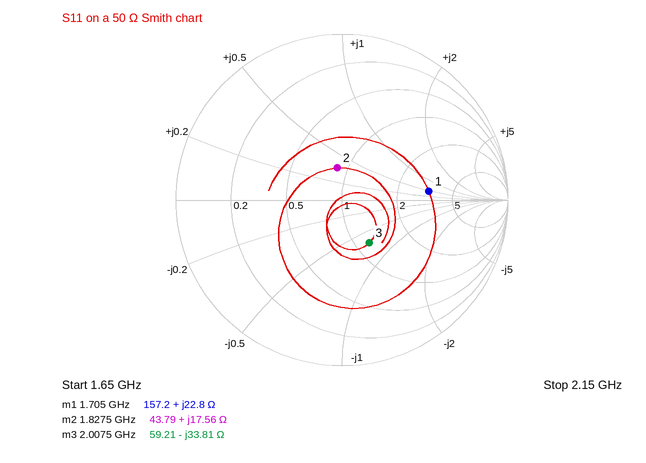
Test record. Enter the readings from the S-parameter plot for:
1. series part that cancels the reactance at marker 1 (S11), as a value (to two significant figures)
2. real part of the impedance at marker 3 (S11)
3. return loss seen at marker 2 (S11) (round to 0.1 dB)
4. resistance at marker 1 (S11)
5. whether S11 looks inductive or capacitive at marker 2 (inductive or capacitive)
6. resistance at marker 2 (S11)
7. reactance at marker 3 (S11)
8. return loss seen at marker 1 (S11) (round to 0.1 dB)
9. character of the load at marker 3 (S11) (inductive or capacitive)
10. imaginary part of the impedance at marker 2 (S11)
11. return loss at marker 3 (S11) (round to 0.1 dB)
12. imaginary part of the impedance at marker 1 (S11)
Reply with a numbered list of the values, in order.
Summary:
1. 4.1 pF
2. 59.21 Ω
3. 14.2 dB
4. 157.2 Ω
5. inductive
6. 43.79 Ω
7. -33.81 Ω
8. 5.6 dB
9. capacitive
10. +17.56 Ω
11. 10.3 dB
12. +22.8 Ω
